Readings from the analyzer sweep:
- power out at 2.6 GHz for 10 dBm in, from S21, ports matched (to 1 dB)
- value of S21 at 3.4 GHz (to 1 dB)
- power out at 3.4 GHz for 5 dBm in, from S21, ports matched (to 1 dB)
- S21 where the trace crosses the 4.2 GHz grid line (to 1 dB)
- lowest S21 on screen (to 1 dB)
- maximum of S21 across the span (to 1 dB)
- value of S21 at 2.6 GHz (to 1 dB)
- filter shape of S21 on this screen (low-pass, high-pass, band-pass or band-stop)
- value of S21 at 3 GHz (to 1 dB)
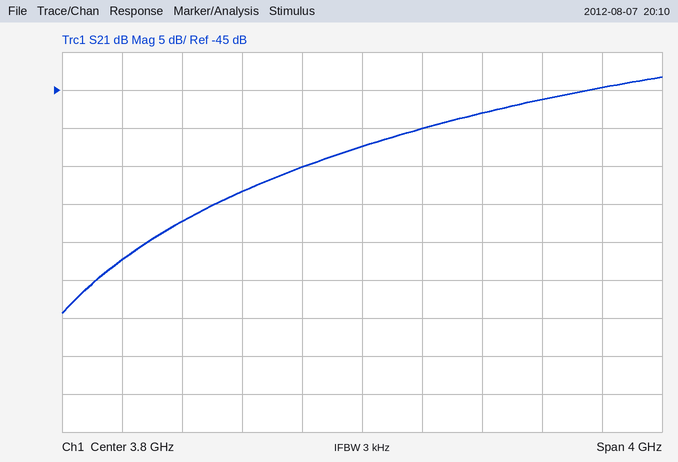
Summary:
-52 dBm
-55 dB
-50 dBm
-50 dB
-74 dB
-43 dB
-62 dB
high-pass
-58 dB
